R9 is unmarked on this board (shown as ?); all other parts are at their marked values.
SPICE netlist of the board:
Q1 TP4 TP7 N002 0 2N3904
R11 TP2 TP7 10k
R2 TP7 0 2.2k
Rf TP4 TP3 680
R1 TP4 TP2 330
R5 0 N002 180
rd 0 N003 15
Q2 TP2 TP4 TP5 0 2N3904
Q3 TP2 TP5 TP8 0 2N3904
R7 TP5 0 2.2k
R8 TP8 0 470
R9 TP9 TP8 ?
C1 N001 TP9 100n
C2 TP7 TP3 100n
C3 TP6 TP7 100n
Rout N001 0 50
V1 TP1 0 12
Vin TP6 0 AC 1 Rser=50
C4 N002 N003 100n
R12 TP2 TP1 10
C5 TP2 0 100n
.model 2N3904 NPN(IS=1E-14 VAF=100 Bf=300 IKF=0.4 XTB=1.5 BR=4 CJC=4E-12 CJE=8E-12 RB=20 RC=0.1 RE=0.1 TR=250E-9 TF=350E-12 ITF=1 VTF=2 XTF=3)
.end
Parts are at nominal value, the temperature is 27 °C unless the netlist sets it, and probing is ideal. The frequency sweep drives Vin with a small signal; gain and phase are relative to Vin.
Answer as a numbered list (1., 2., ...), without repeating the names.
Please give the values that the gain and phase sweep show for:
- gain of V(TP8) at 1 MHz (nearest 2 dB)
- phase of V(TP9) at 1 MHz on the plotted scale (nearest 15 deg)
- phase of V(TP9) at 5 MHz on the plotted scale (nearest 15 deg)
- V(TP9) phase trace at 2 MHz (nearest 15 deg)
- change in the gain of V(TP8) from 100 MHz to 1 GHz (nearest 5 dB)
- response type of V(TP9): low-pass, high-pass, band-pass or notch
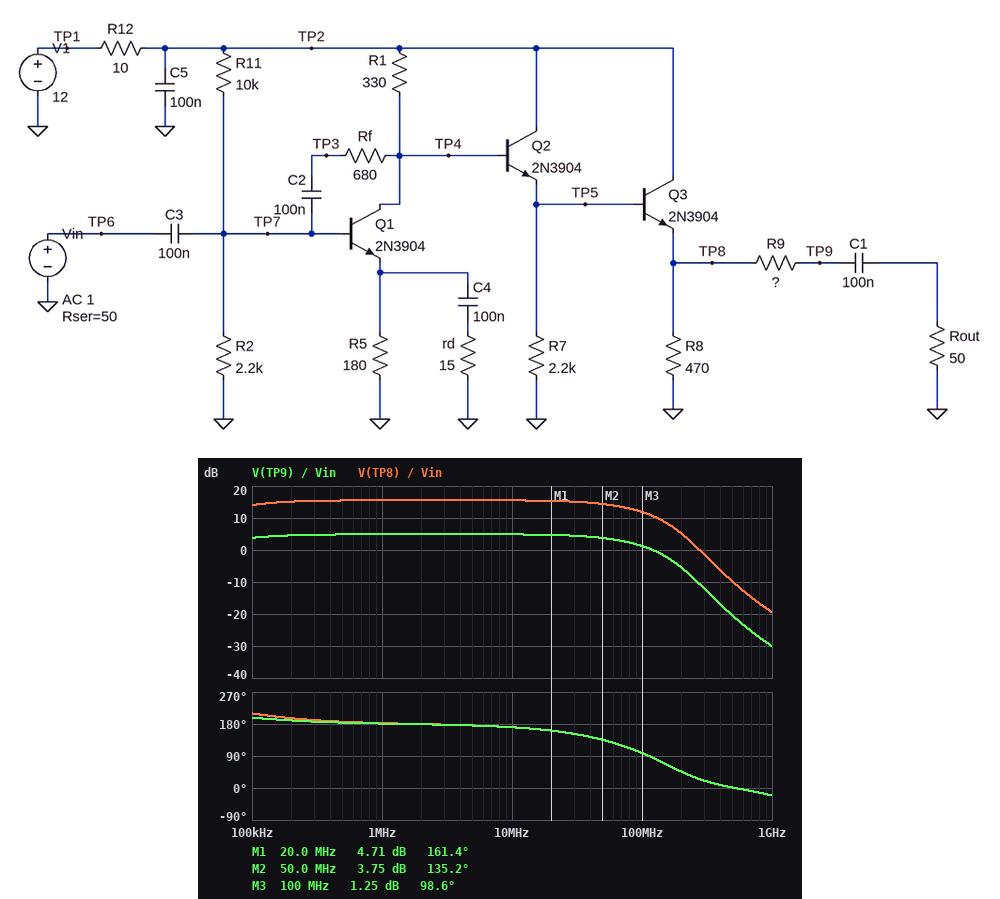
1. 16 dB
2. 180 deg
3. 180 deg
4. 180 deg
5. -30 dB
6. low-pass
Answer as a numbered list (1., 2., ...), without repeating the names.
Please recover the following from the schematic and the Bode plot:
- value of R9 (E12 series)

1. 120 Ω
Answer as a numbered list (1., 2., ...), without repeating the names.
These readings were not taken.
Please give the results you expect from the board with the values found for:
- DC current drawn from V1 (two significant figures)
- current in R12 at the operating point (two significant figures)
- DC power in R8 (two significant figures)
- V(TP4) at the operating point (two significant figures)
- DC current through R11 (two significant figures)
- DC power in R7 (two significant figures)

1. 29 mA
2. 29 mA
3. 130 mW
4. 9.2 V
5. 960 µA
6. 33 mW
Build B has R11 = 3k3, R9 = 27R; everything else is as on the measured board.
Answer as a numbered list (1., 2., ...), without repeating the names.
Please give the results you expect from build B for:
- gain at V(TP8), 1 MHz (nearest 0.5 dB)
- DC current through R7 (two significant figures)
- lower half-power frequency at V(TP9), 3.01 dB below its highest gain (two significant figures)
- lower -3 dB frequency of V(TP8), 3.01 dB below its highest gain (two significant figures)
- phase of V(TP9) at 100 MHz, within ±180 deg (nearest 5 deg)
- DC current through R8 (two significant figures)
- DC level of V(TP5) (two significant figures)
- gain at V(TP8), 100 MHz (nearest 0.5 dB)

1. 15.5 dB
2. 1.8 mA
3. 61 kHz
4. 69 kHz
5. 85 deg
6. 7.0 mA
7. 4.0 V
8. 8.5 dB
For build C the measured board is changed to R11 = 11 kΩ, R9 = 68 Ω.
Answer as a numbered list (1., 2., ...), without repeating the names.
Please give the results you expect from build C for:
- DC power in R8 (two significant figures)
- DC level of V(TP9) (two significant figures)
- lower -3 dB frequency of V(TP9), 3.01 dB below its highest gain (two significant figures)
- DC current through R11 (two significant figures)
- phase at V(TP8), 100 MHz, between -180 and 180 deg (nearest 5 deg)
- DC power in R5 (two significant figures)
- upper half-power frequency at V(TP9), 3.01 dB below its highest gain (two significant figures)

1. 140 mW
2. 8.1 V
3. 50 kHz
4. 890 µA
5. 95 deg
6. 8.1 mW
7. 90 MHz
